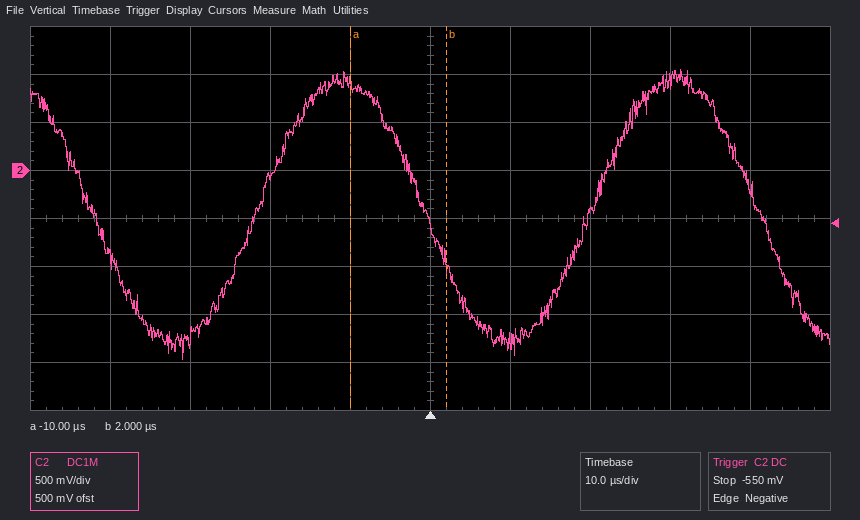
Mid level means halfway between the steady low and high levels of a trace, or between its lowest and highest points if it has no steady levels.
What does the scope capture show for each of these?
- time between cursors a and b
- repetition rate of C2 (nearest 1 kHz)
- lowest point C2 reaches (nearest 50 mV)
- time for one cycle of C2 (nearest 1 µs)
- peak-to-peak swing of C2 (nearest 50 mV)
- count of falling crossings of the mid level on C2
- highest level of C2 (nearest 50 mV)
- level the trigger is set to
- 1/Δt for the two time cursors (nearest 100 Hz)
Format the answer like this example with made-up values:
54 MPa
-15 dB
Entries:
12 µs
24 kHz
-1.95 V
42 µs
3.00 V
3
1.05 V
-550 mV
83.3 kHz
